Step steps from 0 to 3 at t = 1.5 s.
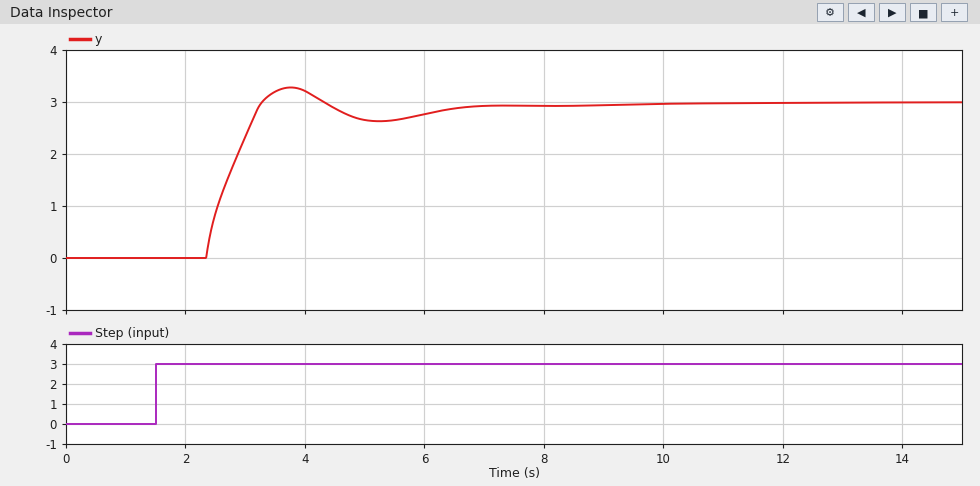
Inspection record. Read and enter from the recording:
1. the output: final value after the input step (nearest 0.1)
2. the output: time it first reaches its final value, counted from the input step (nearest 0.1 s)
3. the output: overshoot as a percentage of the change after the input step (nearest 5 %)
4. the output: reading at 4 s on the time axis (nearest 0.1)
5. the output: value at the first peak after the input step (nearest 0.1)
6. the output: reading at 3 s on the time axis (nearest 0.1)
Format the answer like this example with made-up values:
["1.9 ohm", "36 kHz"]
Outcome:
["3.0", "1.8 s", "10 %", "3.2", "3.3", "2.3"]
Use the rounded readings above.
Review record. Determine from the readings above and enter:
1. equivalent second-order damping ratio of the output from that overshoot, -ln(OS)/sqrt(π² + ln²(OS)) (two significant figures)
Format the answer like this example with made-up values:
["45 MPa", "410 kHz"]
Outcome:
["0.59"]
